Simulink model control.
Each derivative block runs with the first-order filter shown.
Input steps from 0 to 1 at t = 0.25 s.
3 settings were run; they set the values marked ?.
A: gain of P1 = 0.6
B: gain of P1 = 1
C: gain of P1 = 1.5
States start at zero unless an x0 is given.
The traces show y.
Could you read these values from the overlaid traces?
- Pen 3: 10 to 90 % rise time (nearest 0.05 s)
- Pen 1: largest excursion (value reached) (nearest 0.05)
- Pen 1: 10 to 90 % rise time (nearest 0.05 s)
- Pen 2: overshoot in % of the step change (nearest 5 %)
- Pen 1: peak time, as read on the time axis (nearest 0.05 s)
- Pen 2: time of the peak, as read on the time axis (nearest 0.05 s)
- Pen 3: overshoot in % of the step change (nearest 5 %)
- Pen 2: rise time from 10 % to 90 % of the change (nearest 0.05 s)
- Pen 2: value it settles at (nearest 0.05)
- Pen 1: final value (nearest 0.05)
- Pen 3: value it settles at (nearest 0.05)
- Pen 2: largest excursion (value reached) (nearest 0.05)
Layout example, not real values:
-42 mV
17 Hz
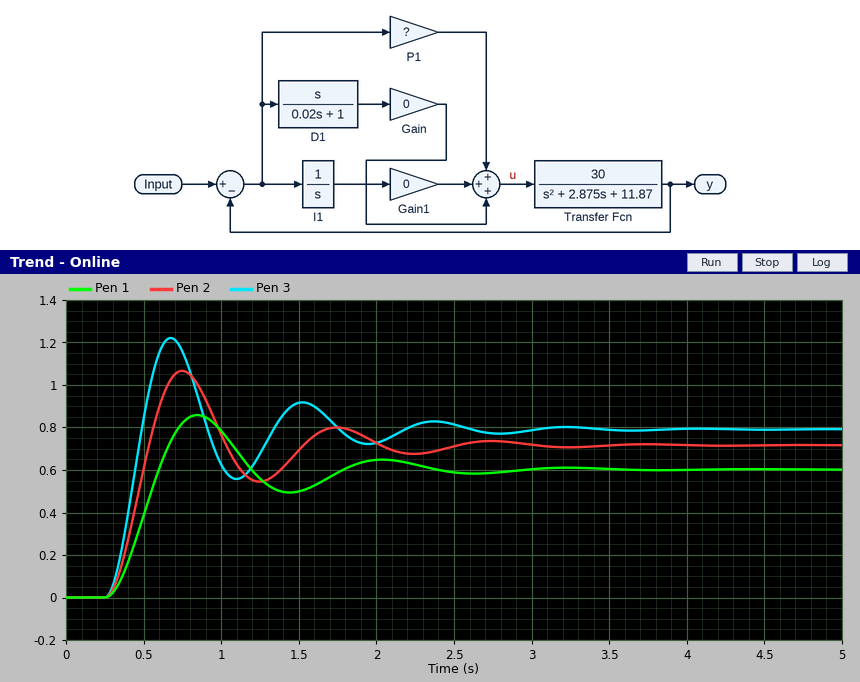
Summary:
0.15 s
0.85
0.25 s
50 %
0.85 s
0.75 s
55 %
0.20 s
0.70
0.60
0.80
1.05
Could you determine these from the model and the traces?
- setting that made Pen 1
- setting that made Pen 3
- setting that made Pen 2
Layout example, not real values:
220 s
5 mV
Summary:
A
C
B
